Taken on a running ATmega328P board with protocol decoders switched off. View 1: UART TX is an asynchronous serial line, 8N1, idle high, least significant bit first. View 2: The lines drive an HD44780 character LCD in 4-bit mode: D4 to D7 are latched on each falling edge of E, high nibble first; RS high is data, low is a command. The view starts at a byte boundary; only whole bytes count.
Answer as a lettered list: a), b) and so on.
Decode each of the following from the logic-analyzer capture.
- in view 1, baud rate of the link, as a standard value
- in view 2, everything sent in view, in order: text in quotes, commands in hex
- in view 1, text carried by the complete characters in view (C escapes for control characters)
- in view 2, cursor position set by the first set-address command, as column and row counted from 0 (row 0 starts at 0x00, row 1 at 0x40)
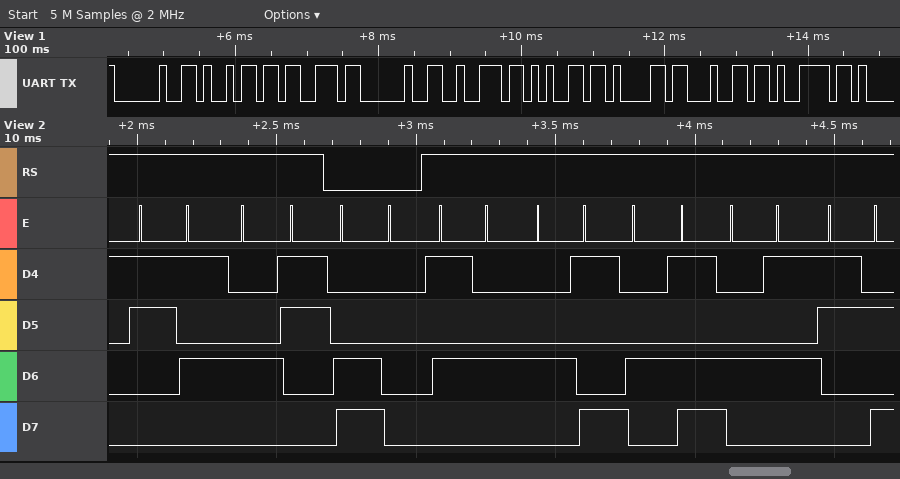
a) 9600 baud
b) "5C" 0xC0 "TIME:"
c) " is ready"
d) column 0, row 1
